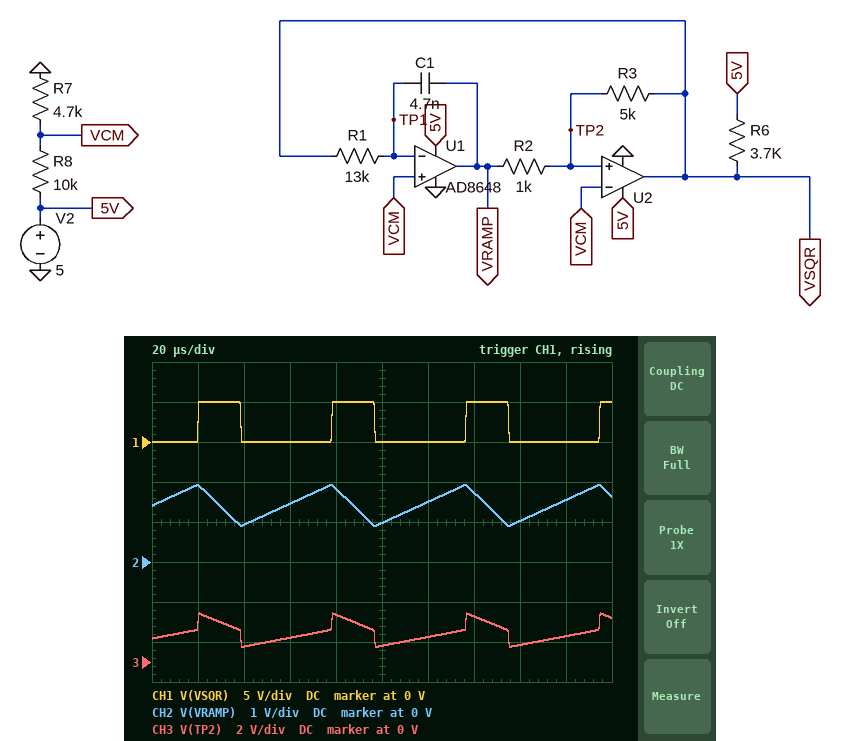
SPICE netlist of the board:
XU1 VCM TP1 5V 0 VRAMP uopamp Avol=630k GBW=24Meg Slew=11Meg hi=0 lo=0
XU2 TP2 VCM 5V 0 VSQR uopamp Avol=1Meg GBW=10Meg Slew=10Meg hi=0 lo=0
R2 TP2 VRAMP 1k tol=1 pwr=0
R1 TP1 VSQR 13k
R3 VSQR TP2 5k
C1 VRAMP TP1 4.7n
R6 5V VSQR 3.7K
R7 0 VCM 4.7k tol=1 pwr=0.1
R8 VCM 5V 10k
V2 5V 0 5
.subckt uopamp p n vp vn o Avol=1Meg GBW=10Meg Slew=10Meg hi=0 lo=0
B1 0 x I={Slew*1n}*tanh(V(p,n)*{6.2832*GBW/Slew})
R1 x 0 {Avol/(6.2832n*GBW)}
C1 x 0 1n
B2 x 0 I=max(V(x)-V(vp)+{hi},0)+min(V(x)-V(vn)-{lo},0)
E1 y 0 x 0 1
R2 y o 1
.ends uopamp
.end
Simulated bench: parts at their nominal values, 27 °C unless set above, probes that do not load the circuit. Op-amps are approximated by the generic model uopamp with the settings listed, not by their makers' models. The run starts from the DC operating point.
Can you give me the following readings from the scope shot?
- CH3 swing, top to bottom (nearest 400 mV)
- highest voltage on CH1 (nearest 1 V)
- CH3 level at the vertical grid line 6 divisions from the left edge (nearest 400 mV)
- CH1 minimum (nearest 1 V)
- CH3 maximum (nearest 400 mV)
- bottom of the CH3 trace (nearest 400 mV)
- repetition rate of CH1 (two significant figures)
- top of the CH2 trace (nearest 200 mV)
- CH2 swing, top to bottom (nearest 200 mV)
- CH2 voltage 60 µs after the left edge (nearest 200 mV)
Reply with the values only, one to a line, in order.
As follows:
1.6 V
5 V
1.2 V
0 V
2.4 V
800 mV
17 kHz
2.0 V
1.0 V
1.4 V
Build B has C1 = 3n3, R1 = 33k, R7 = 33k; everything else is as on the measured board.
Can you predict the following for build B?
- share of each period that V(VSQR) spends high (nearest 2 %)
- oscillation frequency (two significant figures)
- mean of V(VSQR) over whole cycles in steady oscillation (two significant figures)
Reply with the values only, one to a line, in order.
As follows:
76 %
8.0 kHz
3.8 V
